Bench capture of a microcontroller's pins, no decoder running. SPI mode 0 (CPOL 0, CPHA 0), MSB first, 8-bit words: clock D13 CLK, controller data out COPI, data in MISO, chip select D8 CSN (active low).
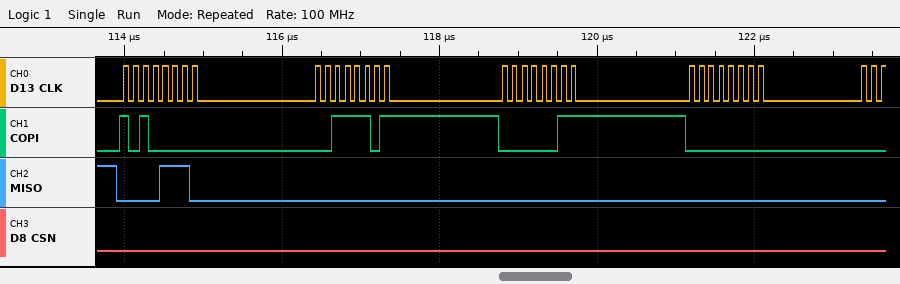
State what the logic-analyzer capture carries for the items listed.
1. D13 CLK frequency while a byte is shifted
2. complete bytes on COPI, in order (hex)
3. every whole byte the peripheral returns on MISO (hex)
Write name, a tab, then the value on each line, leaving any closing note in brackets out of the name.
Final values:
D13 CLK frequency while a byte is shifted	8 MHz
complete bytes on COPI, in order	A0 3D 03 00
every whole byte the peripheral returns on MISO	0E 00 00 00
